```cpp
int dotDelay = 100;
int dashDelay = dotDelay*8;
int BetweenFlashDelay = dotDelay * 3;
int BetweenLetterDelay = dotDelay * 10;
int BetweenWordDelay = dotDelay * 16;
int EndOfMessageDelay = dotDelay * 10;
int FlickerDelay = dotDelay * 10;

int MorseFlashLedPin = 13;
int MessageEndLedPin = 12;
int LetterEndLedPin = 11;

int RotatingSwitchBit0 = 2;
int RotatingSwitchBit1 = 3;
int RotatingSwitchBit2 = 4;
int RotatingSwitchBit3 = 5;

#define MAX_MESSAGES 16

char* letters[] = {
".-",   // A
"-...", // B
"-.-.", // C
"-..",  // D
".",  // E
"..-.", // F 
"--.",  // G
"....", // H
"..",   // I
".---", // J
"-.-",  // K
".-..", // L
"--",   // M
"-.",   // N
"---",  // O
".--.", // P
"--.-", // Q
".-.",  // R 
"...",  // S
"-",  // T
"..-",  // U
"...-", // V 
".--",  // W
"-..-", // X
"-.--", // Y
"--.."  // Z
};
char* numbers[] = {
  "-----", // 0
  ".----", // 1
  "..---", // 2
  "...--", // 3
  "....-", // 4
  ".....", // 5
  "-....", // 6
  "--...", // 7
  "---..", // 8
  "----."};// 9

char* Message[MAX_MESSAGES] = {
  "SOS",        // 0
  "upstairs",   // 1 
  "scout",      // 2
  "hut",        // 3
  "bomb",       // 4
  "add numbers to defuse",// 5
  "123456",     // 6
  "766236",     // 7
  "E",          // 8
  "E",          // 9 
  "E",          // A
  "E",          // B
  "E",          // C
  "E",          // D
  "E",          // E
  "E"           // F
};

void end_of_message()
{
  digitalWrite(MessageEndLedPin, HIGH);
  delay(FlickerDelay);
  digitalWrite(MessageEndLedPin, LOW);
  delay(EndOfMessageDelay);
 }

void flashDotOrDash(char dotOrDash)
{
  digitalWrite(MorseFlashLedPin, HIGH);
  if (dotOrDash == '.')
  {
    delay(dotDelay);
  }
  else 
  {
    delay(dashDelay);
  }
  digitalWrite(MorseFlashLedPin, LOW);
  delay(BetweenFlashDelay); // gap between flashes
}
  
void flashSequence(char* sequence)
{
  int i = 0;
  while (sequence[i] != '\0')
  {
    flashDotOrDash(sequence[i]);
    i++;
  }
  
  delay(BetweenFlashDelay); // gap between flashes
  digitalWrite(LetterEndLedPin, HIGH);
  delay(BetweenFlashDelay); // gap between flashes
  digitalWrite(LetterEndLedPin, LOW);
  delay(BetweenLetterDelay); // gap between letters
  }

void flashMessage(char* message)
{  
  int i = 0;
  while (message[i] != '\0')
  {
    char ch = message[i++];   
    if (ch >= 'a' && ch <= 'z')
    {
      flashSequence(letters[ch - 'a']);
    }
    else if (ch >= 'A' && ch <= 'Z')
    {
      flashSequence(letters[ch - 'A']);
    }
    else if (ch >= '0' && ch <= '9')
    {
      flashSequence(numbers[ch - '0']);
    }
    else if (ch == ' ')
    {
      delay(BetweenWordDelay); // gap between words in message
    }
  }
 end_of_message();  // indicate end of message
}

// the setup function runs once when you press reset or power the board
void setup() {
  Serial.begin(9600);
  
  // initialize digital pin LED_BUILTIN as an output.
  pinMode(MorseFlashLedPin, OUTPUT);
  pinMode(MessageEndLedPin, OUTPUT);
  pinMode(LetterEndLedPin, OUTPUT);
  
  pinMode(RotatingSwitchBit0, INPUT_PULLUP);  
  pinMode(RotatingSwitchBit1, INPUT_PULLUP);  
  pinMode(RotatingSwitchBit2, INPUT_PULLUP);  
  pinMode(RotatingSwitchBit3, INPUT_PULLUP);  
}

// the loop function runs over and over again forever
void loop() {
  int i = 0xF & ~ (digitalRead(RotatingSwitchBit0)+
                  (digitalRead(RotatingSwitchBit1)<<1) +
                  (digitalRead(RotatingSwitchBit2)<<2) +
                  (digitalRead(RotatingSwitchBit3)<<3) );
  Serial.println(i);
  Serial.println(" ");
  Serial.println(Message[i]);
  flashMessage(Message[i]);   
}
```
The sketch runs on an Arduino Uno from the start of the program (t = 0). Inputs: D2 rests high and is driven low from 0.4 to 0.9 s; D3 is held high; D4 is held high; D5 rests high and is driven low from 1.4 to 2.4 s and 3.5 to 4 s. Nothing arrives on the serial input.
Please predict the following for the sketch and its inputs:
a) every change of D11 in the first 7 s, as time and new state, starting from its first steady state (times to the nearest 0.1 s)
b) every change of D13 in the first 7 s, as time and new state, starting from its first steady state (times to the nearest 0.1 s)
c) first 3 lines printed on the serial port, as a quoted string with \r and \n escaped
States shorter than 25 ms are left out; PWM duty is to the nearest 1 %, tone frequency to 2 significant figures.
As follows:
0 s low; 1.5 s high; 1.8 s low; 6.4 s high; 6.7 s low
0 s high; 0.1 s low; 0.4 s high; 0.5 s low; 0.8 s high; 0.9 s low; 2.8 s high; 3.6 s low; 3.9 s high; 4.7 s low; 5 s high; 5.8 s low
"0\r\n \r\nSOS\r\n"
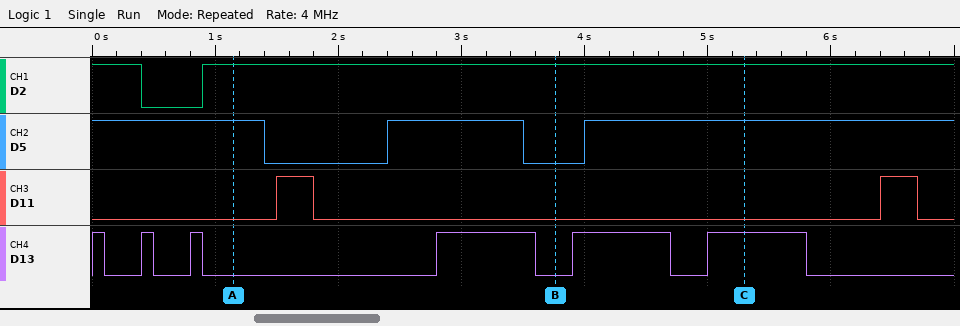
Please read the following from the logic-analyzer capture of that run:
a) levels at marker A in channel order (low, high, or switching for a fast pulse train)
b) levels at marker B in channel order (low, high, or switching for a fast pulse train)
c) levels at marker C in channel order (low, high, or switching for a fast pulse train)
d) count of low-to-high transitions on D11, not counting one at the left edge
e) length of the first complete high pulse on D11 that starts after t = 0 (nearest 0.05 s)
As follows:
D2 high, D5 high, D11 low, D13 low
D2 high, D5 low, D11 low, D13 low
D2 high, D5 high, D11 low, D13 high
2
0.30 s
